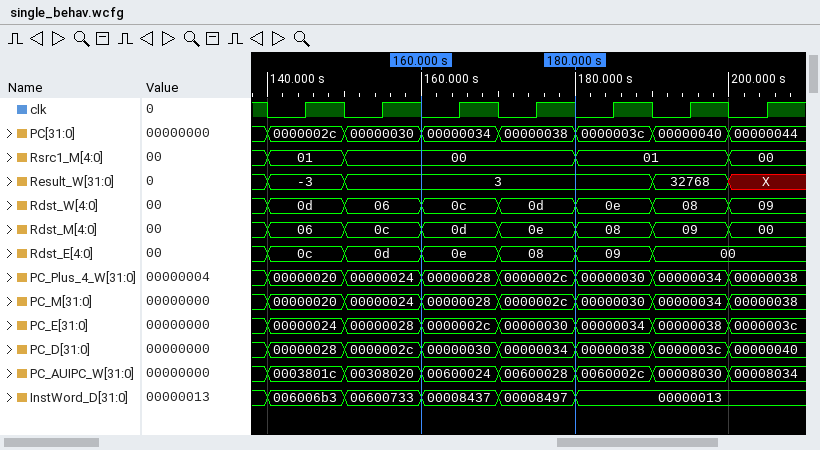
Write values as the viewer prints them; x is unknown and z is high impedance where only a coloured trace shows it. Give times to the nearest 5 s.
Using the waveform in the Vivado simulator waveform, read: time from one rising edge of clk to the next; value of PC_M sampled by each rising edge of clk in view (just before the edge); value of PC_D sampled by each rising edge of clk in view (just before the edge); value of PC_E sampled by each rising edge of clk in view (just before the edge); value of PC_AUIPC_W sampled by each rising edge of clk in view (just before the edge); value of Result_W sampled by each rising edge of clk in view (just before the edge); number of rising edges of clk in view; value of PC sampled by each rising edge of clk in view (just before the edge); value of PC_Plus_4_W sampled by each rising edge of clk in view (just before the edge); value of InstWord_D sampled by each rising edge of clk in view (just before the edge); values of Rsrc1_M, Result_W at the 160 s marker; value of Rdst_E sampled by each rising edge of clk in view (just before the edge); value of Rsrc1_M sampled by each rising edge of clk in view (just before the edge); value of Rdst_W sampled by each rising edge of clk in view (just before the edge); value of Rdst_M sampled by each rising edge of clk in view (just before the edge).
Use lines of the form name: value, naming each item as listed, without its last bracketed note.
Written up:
time from one rising edge of clk to the next: 10 s
value of PC_M sampled by each rising edge of clk in view: 00000020, 00000024, 00000028, 0000002c, 00000030, 00000034, 00000038
value of PC_D sampled by each rising edge of clk in view: 00000028, 0000002c, 00000030, 00000034, 00000038, 0000003c, 00000040
value of PC_E sampled by each rising edge of clk in view: 00000024, 00000028, 0000002c, 00000030, 00000034, 00000038, 0000003c
value of PC_AUIPC_W sampled by each rising edge of clk in view: 0003801c, 00308020, 00600024, 00600028, 0060002c, 00008030, 00008034
value of Result_W sampled by each rising edge of clk in view: -3, 3, 3, 3, 3, 32768, X
number of rising edges of clk in view: 7
value of PC sampled by each rising edge of clk in view: 0000002c, 00000030, 00000034, 00000038, 0000003c, 00000040, 00000044
value of PC_Plus_4_W sampled by each rising edge of clk in view: 00000020, 00000024, 00000028, 0000002c, 00000030, 00000034, 00000038
value of InstWord_D sampled by each rising edge of clk in view: 006006b3, 00600733, 00008437, 00008497, 00000013, 00000013, 00000013
values of Rsrc1_M, Result_W at the 160 s marker: Rsrc1_M=00, Result_W=3
value of Rdst_E sampled by each rising edge of clk in view: 0c, 0d, 0e, 08, 09, 00, 00
value of Rsrc1_M sampled by each rising edge of clk in view: 01, 00, 00, 00, 01, 01, 00
value of Rdst_W sampled by each rising edge of clk in view: 0d, 06, 0c, 0d, 0e, 08, 09
value of Rdst_M sampled by each rising edge of clk in view: 06, 0c, 0d, 0e, 08, 09, 00
